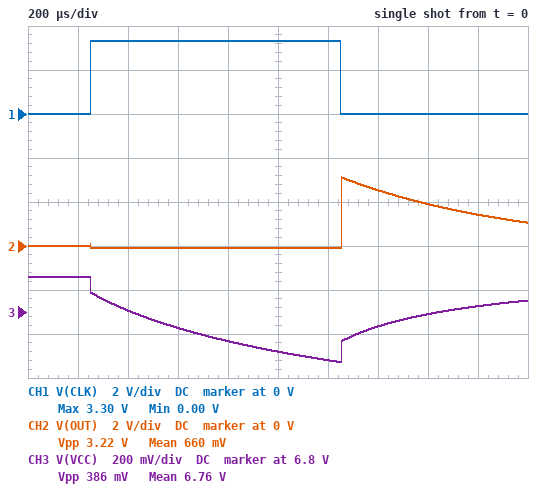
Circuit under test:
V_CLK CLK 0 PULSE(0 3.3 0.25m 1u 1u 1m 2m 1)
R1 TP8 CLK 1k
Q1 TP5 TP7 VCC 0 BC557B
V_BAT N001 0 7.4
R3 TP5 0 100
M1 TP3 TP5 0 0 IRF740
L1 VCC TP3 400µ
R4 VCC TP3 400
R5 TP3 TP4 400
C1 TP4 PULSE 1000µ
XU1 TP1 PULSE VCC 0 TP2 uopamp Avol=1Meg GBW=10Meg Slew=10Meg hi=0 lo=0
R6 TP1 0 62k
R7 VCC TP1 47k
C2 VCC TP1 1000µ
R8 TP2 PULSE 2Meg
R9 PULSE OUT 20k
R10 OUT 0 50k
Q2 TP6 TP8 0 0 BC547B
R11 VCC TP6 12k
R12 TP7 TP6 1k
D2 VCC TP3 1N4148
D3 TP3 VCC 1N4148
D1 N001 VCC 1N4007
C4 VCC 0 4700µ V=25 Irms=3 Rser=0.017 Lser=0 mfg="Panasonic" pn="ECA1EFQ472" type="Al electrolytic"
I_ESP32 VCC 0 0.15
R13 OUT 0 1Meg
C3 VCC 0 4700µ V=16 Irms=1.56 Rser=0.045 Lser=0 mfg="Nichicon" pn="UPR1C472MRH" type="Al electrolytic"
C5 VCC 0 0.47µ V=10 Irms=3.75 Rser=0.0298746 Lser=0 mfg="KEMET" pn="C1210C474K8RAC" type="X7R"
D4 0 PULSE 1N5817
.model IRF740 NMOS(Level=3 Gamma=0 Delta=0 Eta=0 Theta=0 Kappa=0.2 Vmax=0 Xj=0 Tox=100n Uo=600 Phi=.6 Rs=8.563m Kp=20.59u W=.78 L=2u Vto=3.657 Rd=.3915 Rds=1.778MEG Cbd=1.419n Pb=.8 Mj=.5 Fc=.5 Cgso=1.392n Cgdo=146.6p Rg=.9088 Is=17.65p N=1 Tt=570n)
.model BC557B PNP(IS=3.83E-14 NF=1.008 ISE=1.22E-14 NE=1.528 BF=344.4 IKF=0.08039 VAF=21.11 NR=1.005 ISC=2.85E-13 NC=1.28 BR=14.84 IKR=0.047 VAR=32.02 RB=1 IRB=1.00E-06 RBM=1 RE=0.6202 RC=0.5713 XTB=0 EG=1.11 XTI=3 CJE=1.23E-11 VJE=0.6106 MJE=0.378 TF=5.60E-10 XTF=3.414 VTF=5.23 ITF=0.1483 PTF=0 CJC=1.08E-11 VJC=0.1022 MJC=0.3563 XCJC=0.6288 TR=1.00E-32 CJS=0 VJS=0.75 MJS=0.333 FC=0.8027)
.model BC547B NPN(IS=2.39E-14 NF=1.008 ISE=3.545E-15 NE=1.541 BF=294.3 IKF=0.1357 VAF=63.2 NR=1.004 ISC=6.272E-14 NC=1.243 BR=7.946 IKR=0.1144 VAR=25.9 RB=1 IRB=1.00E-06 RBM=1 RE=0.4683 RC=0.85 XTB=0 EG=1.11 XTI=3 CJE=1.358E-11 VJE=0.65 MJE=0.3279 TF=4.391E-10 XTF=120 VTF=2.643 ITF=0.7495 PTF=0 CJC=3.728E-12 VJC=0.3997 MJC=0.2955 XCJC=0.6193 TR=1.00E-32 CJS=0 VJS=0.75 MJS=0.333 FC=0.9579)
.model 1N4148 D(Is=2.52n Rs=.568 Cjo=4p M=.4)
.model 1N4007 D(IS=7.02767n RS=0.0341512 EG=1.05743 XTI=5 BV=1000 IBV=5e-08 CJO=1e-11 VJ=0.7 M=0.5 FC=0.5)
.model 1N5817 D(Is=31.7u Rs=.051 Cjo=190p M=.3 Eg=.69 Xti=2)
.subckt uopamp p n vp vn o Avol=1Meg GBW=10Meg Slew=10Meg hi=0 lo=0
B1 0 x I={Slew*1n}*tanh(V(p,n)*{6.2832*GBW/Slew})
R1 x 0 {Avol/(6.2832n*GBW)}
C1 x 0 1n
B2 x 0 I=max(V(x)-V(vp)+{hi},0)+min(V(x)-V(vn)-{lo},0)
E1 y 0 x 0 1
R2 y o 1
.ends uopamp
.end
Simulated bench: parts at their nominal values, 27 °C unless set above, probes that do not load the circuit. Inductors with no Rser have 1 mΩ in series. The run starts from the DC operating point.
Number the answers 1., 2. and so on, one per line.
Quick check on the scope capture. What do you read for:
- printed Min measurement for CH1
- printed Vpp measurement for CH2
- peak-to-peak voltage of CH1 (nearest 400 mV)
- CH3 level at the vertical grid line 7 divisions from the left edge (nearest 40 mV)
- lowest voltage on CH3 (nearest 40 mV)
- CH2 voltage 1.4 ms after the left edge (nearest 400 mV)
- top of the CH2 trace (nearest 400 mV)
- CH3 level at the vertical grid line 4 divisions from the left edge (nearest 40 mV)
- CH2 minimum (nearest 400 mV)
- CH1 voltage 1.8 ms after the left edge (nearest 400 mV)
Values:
1. 0.00 V
2. 3.22 V
3. 3.2 V
4. 6.72 V
5. 6.56 V
6. 2.4 V
7. 3.2 V
8. 6.68 V
9. 0 V
10. 0 V
